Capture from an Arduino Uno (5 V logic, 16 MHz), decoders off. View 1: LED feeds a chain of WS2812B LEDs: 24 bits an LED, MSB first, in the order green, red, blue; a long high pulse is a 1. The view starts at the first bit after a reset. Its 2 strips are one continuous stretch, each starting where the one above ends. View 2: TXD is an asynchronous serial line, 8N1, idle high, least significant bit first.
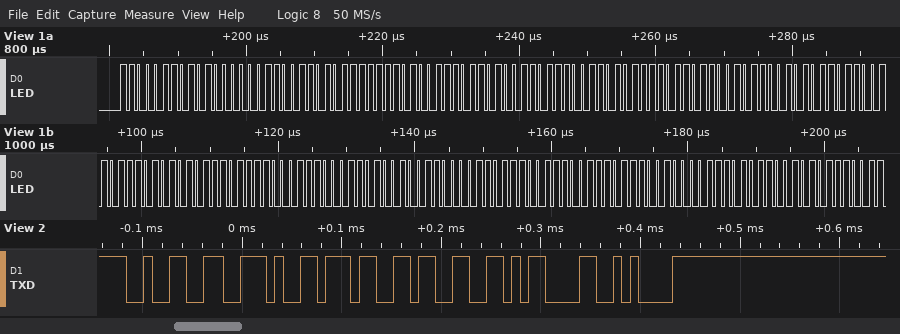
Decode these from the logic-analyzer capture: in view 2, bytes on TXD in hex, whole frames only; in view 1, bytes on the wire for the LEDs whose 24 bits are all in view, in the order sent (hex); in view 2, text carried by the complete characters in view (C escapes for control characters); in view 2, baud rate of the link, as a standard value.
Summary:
32 2E 37 33 0D 0A
C6 A0 66 BF A7 69 B9 AF 6C B2 B6 6E AB BC 71 A4 C3 73 9D C8 75
"2.73\r\n"
115200 baud
